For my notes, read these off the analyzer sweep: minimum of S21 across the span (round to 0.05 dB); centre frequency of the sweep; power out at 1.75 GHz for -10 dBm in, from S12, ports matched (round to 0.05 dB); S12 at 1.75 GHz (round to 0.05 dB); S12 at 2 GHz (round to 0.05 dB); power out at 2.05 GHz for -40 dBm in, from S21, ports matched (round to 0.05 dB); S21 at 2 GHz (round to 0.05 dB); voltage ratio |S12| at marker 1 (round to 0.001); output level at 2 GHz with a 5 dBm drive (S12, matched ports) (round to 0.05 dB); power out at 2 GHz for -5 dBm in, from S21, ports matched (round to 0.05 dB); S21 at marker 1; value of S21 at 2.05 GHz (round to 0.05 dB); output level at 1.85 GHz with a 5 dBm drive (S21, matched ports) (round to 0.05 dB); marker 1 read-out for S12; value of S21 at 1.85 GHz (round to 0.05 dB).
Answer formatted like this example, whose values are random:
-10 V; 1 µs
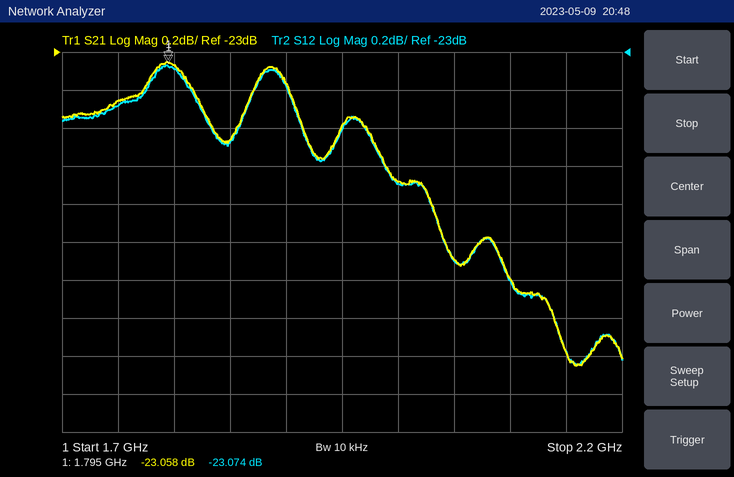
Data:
-24.65 dB; 1.95 GHz; -33.30 dBm; -23.30 dB; -23.70 dB; -64.10 dBm; -23.70 dB; 0.070; -18.70 dBm; -28.70 dBm; -23.058 dB; -24.10 dB; -18.45 dBm; -23.074 dB; -23.45 dB
